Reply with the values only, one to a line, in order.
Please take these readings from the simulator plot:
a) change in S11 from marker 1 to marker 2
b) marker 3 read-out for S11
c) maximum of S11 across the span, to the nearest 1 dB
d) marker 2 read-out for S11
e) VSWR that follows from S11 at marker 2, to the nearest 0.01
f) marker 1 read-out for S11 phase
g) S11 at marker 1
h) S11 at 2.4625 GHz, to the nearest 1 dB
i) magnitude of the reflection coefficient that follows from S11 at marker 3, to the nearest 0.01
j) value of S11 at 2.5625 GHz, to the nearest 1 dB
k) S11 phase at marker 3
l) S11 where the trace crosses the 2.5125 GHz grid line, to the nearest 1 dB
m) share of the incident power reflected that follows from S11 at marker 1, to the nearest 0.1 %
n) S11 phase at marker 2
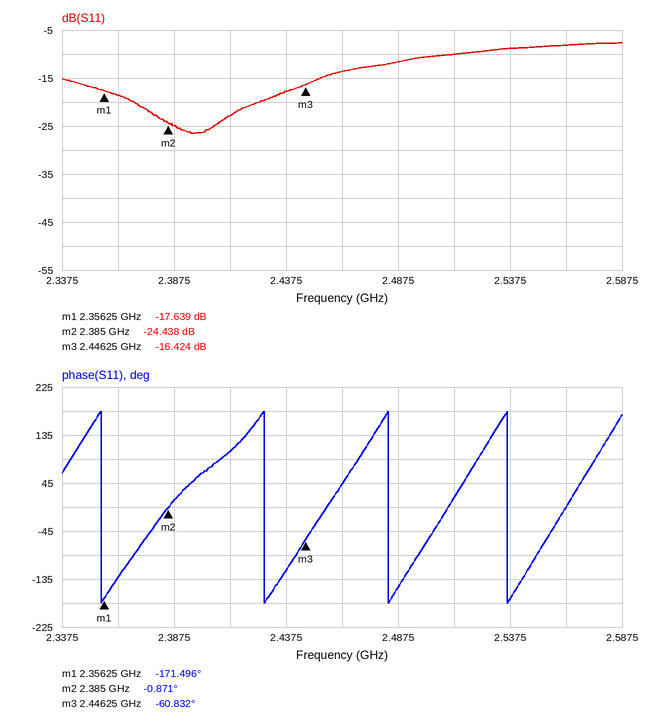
-6.799 dB
-16.424 dB
-8 dB
-24.438 dB
1.13
-171.496°
-17.639 dB
-14 dB
0.15
-8 dB
-60.832°
-10 dB
1.7 %
-0.871°
